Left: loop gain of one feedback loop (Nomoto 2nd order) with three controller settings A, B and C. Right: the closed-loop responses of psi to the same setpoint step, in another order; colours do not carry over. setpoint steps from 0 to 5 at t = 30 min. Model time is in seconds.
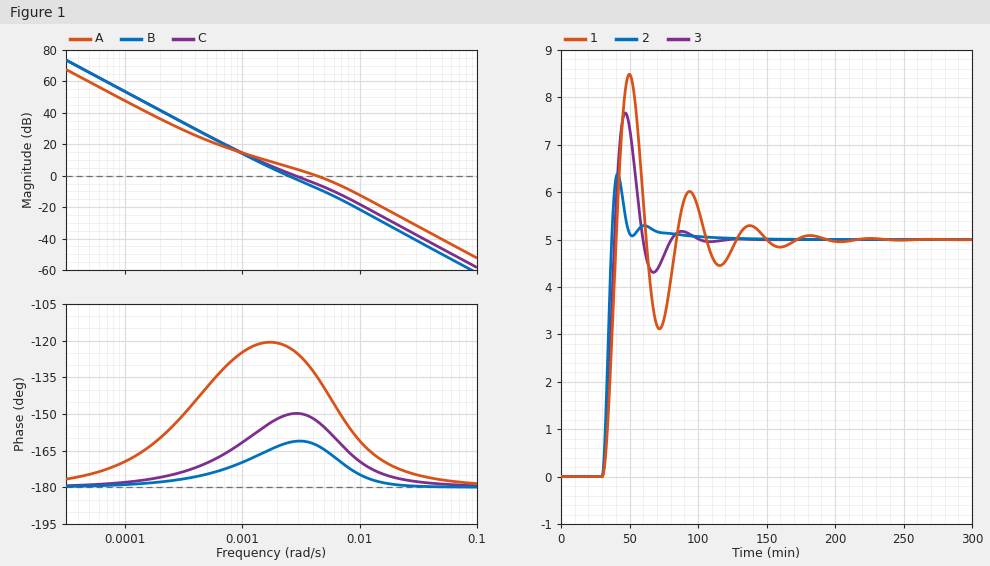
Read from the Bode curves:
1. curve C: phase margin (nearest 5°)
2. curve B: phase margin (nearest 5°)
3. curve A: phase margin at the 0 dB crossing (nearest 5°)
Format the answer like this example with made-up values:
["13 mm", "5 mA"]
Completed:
["30°", "20°", "45°"]
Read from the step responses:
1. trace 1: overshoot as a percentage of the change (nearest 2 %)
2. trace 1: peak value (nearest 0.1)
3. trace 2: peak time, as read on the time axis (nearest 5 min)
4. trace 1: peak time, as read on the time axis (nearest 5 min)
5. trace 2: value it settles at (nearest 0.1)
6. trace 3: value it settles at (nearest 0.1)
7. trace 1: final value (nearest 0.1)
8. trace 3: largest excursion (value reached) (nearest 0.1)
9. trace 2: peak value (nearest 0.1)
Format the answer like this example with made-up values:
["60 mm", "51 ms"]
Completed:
["70 %", "8.5", "40 min", "50 min", "5.0", "5.0", "5.0", "7.7", "6.4"]
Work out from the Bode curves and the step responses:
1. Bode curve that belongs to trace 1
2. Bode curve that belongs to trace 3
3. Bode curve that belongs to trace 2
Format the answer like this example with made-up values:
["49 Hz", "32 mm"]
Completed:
["B", "C", "A"]
